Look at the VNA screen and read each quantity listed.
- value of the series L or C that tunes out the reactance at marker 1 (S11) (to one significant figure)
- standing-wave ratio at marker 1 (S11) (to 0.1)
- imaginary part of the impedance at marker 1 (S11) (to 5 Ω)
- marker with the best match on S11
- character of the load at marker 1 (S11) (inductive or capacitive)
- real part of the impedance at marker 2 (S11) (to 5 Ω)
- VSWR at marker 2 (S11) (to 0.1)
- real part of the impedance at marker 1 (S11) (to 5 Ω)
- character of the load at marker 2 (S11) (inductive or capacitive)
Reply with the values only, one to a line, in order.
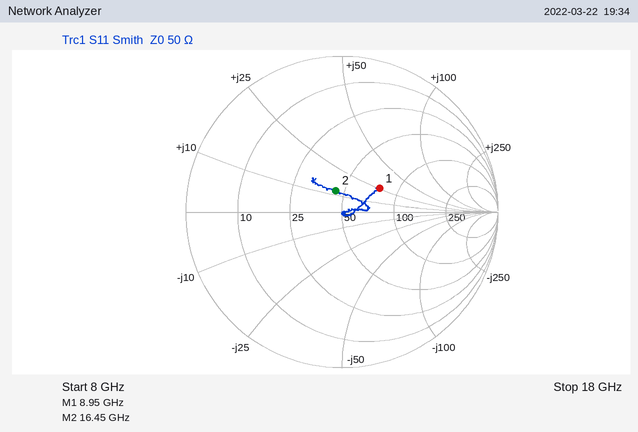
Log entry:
700 fF
1.8
+25 Ω
marker 2
inductive
45 Ω
1.3
75 Ω
inductive
